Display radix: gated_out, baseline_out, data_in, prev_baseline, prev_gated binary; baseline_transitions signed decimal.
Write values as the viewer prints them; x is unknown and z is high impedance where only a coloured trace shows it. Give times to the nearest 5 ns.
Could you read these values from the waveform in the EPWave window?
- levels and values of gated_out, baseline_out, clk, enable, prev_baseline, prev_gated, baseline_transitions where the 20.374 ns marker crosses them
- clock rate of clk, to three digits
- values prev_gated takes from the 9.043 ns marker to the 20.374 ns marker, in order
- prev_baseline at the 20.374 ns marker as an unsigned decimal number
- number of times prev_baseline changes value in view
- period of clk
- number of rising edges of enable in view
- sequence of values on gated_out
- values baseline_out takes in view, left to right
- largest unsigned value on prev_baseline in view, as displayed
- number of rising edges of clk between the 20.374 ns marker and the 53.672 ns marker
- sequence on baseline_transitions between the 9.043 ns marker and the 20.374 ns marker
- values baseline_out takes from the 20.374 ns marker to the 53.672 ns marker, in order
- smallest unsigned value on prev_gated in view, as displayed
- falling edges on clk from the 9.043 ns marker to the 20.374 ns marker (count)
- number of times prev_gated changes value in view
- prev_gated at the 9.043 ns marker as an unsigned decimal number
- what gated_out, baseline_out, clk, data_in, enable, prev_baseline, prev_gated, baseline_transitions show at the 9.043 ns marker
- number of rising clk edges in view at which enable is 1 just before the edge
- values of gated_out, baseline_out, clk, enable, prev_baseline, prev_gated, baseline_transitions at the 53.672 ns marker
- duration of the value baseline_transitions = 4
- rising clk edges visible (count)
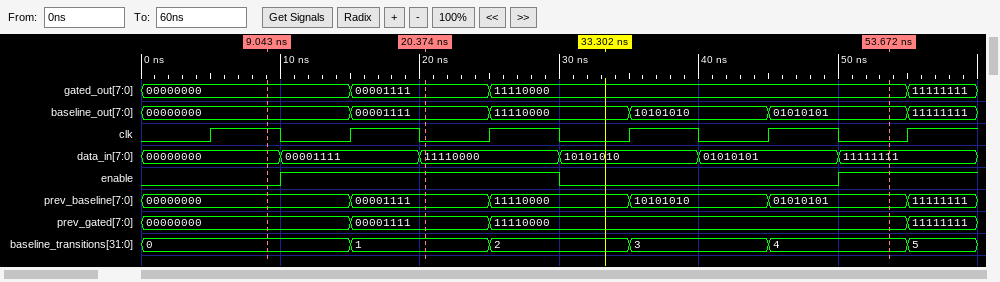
gated_out=00001111, baseline_out=00001111, clk=0, enable=1, prev_baseline=00001111, prev_gated=00001111, baseline_transitions=1
100 MHz
00000000, 00001111
15
5
10 ns
2
00000000, 00001111, 11110000, 11111111
00000000, 00001111, 11110000, 10101010, 01010101, 11111111
11111111
3
0, 1
00001111, 11110000, 10101010, 01010101
00000000
2
3
0
gated_out=00000000, baseline_out=00000000, clk=1, data_in=00000000, enable=0, prev_baseline=00000000, prev_gated=00000000, baseline_transitions=0
3
gated_out=11110000, baseline_out=01010101, clk=0, enable=1, prev_baseline=01010101, prev_gated=11110000, baseline_transitions=4
10 ns
6
